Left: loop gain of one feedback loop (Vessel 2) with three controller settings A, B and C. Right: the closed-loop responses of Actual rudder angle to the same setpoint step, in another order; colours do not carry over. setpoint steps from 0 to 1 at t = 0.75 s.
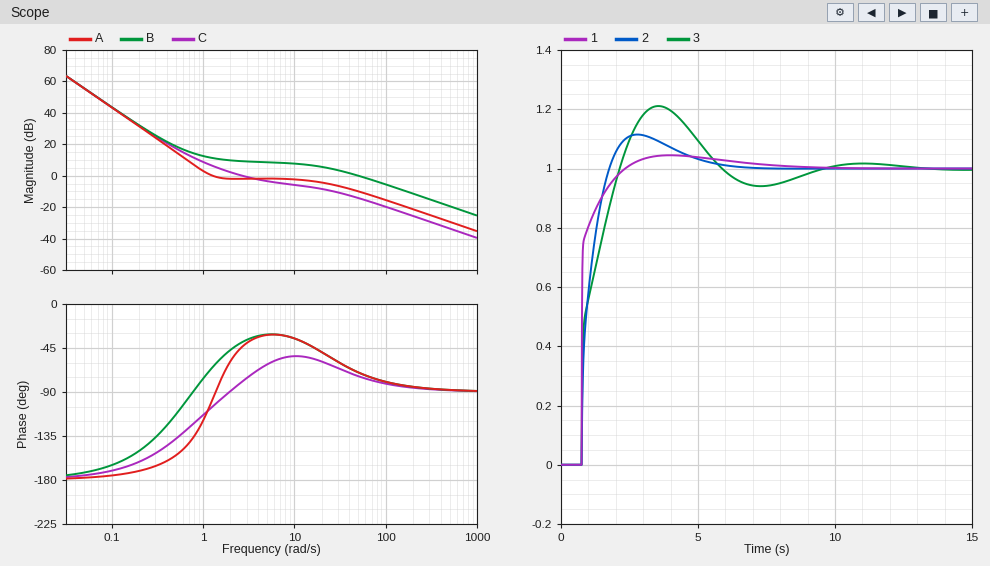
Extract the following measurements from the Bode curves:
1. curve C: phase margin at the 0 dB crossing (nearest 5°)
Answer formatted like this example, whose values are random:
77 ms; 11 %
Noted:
100°
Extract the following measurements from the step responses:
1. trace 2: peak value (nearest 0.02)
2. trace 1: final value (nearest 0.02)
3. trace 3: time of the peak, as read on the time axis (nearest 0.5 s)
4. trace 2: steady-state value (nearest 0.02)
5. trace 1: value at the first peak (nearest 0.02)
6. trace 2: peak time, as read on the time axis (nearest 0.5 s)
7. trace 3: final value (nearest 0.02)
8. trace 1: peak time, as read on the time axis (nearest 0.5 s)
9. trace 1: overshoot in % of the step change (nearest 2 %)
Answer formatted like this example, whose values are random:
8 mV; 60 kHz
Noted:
1.12; 1.00; 3.5 s; 1.00; 1.04; 3.0 s; 1.00; 4.0 s; 4 %
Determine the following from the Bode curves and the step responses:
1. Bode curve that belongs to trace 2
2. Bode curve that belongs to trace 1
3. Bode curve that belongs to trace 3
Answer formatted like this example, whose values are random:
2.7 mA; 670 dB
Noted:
C; B; A
